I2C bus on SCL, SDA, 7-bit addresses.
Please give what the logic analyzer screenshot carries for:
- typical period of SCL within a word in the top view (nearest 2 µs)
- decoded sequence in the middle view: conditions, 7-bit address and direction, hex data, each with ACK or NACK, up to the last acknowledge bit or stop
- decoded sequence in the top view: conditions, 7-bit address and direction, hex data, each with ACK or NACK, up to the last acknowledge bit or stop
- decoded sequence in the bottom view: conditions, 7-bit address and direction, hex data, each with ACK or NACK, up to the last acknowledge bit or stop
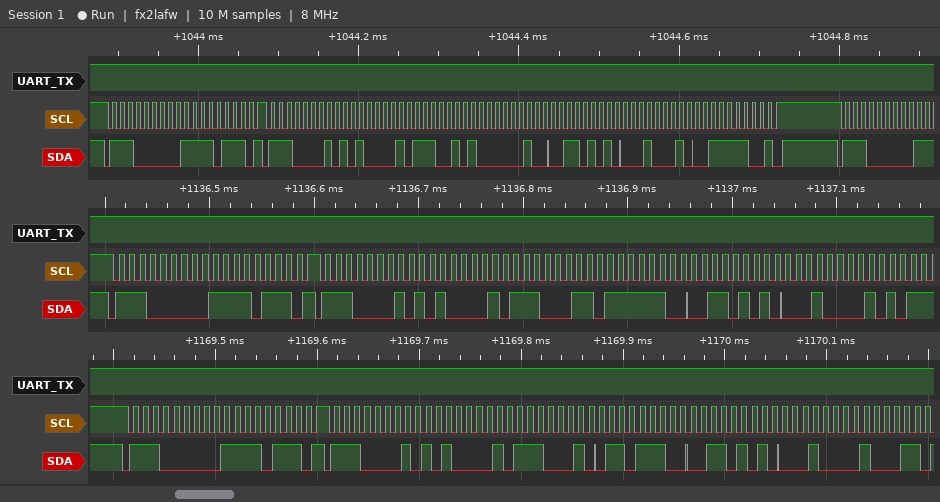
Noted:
10 µs
start, address 70 write ACK, F7 ACK, repeated start, address 70 read ACK, A1 ACK, E3 ACK, FC ACK, 6A ACK, 21 ACK
start, address 70 write ACK, F7 ACK, repeated start, address 70 read ACK, A1 ACK, E5 ACK, 04 ACK, 6A ACK, 22 ACK, 7C NACK, stop, start, address 70 write ACK
start, address 70 write ACK, F7 ACK, repeated start, address 70 read ACK, A1 ACK, E2 ACK, DC ACK, 6A ACK, 21 ACK
